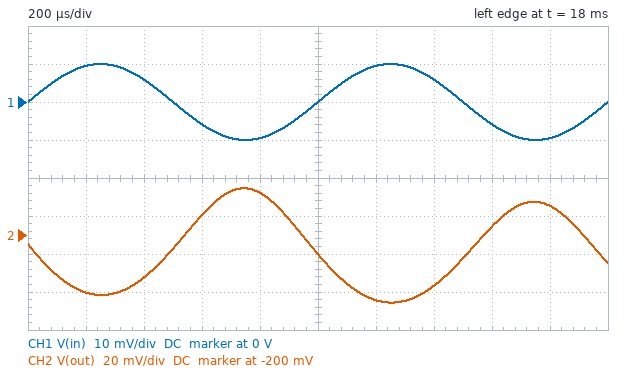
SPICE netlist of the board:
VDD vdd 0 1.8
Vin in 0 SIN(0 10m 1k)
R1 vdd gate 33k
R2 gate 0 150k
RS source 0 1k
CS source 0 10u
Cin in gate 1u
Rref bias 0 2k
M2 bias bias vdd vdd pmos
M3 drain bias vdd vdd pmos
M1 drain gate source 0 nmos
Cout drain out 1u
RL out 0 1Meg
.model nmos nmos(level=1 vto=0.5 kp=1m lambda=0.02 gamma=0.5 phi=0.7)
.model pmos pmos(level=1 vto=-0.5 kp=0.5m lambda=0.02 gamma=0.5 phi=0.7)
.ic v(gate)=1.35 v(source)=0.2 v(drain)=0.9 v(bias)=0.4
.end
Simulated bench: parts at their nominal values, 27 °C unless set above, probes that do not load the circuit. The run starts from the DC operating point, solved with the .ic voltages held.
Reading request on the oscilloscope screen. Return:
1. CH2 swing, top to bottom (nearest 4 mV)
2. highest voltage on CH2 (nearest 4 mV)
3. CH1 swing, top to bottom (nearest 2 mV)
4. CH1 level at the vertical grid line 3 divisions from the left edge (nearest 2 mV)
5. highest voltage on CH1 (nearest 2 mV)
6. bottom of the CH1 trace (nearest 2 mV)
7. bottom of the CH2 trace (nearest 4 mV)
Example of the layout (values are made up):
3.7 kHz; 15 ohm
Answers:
60 mV; -176 mV; 20 mV; -6 mV; 10 mV; -10 mV; -236 mV
